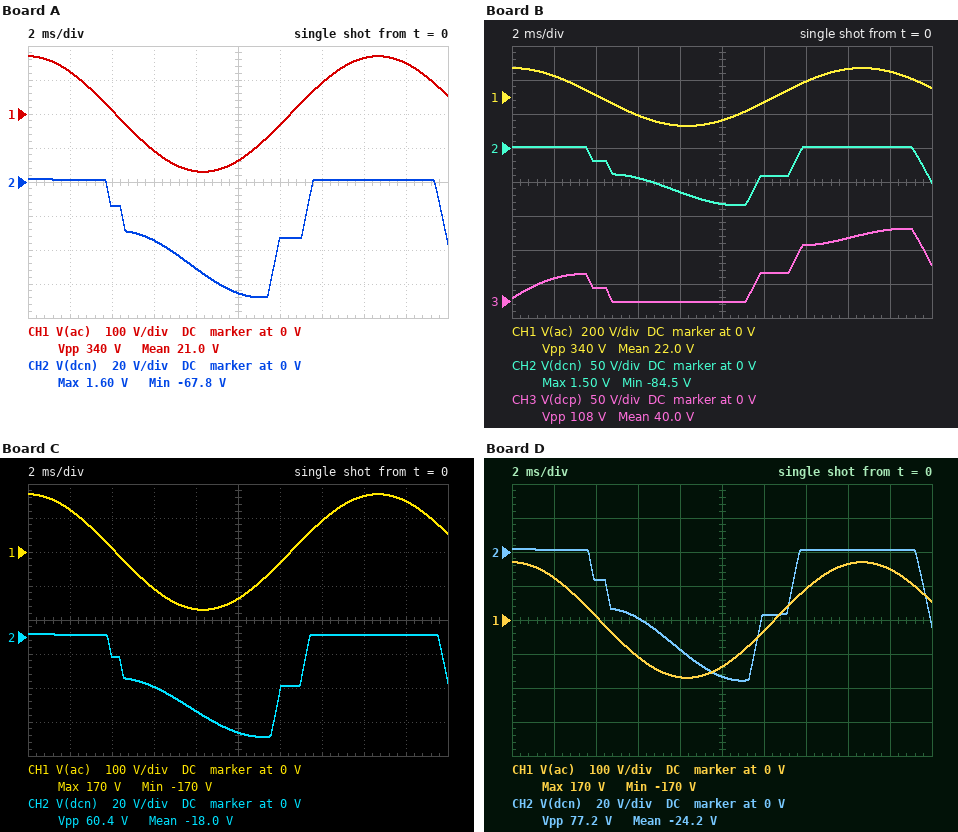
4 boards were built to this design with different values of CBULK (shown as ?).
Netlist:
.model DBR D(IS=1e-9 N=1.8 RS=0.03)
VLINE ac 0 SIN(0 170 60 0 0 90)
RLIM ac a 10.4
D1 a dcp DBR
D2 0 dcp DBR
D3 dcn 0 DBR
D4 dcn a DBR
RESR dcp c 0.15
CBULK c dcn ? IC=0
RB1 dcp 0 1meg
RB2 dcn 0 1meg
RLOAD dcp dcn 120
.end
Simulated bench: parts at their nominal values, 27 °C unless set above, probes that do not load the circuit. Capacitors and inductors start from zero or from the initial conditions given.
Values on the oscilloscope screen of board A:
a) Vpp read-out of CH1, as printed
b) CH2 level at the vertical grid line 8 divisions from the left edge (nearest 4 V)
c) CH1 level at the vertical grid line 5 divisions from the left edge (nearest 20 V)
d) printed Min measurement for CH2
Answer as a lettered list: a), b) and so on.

a) 340 V
b) 0 V
c) -140 V
d) -67.8 V
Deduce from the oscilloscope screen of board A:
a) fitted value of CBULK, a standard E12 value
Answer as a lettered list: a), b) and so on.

a) 1.2 mF
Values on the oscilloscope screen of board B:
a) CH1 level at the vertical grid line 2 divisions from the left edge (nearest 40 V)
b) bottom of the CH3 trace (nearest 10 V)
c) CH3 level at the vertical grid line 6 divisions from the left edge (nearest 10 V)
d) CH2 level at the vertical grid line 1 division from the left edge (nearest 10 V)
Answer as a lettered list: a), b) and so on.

a) 0 V
b) 0 V
c) 40 V
d) 0 V
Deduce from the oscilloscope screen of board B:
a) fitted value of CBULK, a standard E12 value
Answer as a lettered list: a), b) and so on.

a) 820 µF
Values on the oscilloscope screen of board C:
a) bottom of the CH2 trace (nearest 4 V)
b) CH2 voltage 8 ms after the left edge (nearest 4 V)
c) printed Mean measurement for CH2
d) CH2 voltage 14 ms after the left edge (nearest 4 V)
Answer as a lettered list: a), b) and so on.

a) -60 V
b) -44 V
c) -18.0 V
d) 0 V
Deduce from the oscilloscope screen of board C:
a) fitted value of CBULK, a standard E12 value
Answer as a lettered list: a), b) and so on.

a) 1.5 mF
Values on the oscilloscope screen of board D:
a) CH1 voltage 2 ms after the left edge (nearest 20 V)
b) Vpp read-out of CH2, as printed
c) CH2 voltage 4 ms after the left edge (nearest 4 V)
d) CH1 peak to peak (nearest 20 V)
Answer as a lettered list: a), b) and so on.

a) 120 V
b) 77.2 V
c) -16 V
d) 340 V
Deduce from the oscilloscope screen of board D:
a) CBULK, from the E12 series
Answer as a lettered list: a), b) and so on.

a) 1 mF
